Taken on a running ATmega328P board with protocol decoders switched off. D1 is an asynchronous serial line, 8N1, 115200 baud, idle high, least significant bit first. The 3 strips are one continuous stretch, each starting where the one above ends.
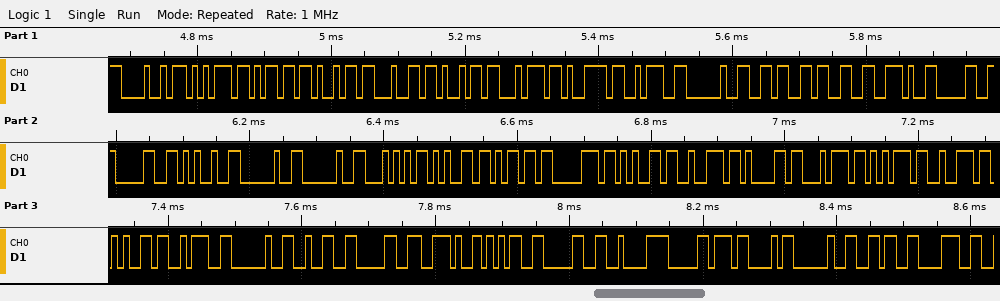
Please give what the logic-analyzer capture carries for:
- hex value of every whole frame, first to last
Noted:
48 75 6D 69 64 69 74 79 3A 20 36 33 2E 30 30 25 20 20 54 65 6D 70 65 72 61 74 75 72 65 3A 20 32 30 2E 35 30 C2 B0 43 20 36 38
